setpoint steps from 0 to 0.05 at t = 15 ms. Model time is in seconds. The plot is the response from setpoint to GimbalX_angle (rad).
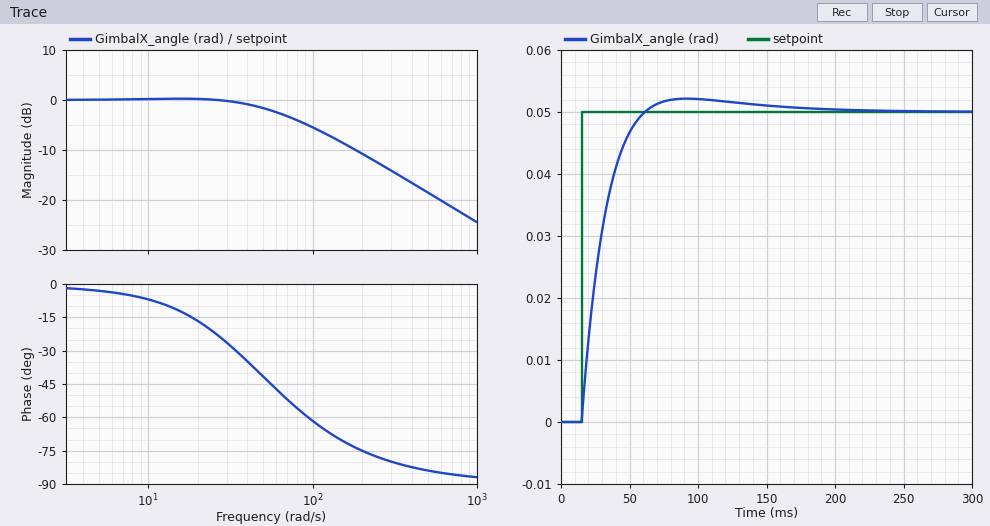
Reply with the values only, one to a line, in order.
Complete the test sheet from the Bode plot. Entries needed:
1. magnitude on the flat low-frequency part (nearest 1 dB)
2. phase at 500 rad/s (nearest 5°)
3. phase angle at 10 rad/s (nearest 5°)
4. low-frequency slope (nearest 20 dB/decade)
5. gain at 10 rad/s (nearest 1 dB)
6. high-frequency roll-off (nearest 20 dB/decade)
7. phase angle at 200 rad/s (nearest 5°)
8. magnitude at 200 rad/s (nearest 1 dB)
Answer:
0 dB
-85°
-5°
0 dB/decade
0 dB
-20 dB/decade
-75°
-11 dB
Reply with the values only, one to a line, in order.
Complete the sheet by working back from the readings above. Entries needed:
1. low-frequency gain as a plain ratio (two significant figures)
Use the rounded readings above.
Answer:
1.0
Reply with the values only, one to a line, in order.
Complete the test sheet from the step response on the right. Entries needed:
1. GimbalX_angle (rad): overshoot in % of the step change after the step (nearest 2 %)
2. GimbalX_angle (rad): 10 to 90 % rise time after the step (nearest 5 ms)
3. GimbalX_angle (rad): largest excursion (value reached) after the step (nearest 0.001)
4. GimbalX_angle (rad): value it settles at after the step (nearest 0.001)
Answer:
4 %
30 ms
0.052
0.050
